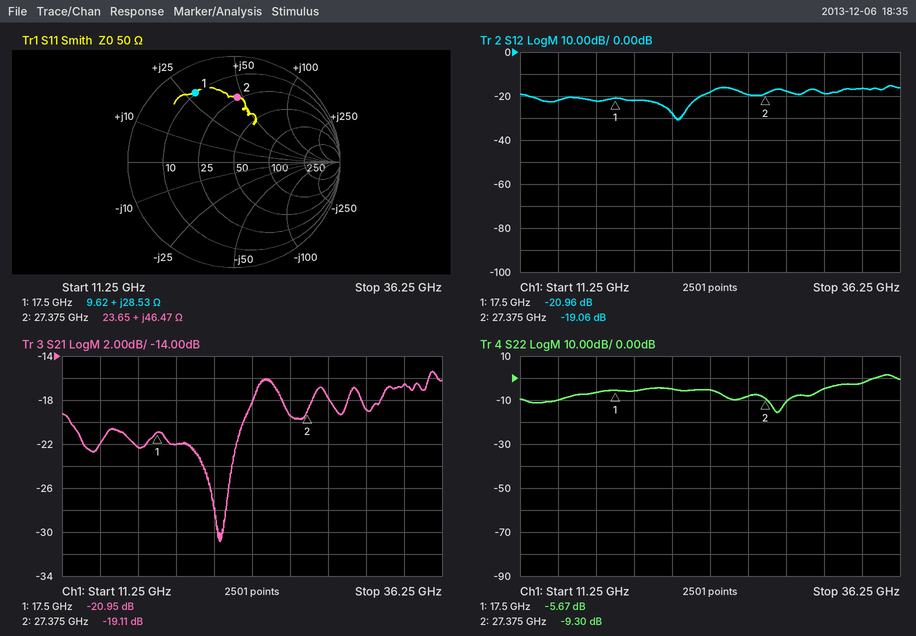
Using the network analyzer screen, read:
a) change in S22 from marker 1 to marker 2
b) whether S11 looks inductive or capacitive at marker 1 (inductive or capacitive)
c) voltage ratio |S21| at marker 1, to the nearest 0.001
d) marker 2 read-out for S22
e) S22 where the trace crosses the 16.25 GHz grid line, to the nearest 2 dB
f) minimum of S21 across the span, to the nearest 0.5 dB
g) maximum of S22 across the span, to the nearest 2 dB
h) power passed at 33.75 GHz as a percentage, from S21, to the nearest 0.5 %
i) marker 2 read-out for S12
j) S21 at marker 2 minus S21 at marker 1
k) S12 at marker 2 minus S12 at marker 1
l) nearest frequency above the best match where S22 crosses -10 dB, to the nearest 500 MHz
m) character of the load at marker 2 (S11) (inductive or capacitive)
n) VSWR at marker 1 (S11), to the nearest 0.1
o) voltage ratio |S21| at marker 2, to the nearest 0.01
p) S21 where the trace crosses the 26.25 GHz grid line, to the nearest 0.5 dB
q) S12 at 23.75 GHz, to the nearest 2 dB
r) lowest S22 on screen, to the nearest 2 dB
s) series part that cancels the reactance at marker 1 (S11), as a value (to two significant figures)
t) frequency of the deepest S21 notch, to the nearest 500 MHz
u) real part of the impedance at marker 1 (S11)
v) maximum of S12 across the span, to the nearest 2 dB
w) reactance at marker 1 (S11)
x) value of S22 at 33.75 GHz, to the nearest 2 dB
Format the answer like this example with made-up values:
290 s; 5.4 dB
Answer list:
-3.63 dB; inductive; 0.090; -9.30 dB; -6 dB; -31.0 dB; 2 dB; 2.0 %; -19.06 dB; 1.84 dB; 1.90 dB; 29.0 GHz; inductive; 6.9; 0.11; -19.5 dB; -18 dB; -16 dB; 320 fF; 21.5 GHz; 9.62 Ω; -16 dB; +28.53 Ω; -2 dB
